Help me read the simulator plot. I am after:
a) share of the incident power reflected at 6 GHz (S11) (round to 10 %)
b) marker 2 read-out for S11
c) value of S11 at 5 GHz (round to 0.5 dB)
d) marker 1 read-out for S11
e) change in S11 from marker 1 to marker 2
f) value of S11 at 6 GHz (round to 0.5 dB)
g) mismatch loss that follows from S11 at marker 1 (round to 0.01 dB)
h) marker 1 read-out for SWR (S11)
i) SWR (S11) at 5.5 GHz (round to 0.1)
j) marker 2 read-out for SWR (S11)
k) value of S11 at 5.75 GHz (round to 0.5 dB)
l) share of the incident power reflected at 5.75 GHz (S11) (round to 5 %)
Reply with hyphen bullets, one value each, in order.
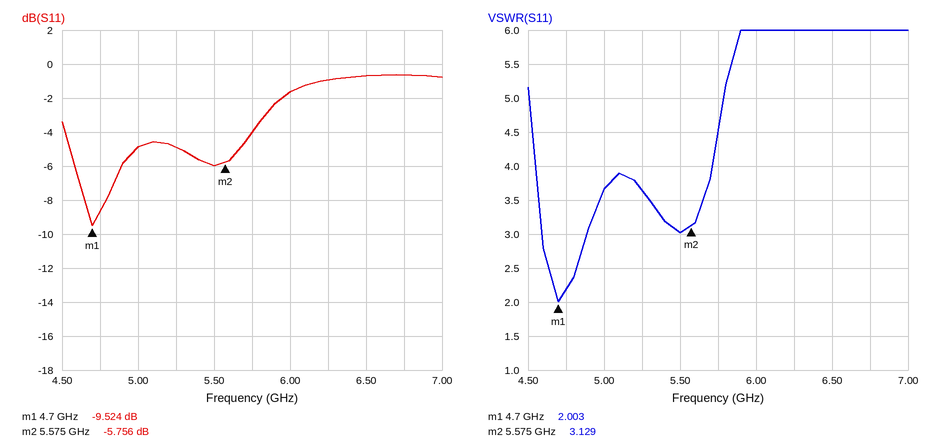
- 70 %
- -5.756 dB
- -5.0 dB
- -9.524 dB
- 3.768 dB
- -1.5 dB
- 0.51 dB
- 2.003
- 3.0
- 3.129
- -4.0 dB
- 40 %
